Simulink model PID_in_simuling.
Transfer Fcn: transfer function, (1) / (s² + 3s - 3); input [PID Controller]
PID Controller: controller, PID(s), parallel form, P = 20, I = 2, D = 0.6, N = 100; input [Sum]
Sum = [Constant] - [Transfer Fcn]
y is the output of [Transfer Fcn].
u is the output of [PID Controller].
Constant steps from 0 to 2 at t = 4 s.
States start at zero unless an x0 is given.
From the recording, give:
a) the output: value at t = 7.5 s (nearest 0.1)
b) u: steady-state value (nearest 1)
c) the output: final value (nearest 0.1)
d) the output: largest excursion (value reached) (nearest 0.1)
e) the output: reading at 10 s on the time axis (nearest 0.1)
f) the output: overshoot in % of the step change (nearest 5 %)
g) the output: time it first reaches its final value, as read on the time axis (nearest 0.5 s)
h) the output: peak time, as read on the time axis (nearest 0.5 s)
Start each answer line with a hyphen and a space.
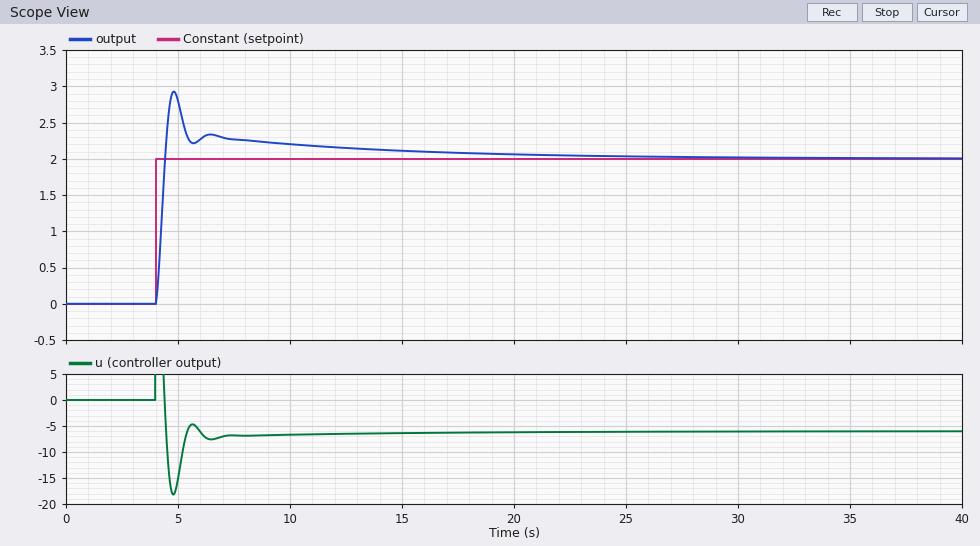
- 2.3
- -6
- 2.0
- 2.9
- 2.2
- 45 %
- 4.5 s
- 5.0 s
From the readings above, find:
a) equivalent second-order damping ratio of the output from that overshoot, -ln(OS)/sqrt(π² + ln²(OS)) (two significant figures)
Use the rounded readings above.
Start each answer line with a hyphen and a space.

- 0.25
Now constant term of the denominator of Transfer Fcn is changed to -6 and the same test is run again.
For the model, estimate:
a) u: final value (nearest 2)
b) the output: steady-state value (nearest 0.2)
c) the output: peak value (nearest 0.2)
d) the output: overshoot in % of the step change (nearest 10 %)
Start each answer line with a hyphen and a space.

- -12
- 2.0
- 3.4
- 70 %
